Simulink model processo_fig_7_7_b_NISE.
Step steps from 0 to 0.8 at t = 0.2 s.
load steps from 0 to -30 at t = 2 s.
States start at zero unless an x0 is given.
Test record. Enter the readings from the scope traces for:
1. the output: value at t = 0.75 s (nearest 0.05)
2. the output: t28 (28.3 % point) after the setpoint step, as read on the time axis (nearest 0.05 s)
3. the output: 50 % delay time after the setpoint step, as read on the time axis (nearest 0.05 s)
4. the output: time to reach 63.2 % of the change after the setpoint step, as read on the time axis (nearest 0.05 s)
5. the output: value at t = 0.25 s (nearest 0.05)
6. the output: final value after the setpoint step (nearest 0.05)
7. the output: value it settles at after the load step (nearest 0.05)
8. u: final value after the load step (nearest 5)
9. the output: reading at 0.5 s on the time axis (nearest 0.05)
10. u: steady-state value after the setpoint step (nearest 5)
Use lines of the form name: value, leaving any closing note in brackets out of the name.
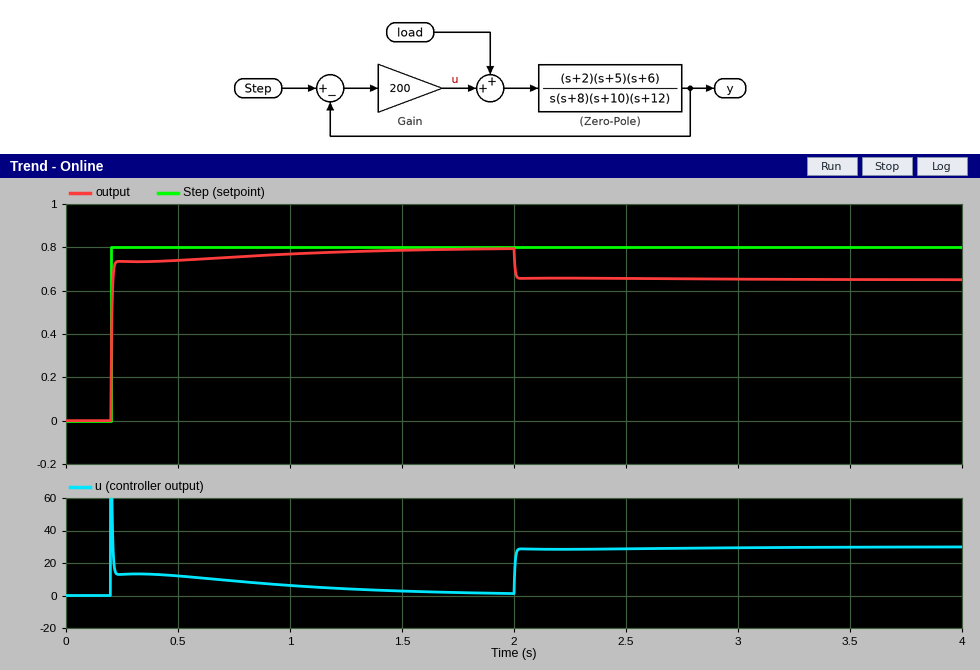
the output: value at t = 0.75 s: 0.75
the output: t28 (28.3 % point) after the setpoint step, as read on the time axis: 0.20 s
the output: 50 % delay time after the setpoint step, as read on the time axis: 0.20 s
the output: time to reach 63.2 % of the change after the setpoint step, as read on the time axis: 0.20 s
the output: value at t = 0.25 s: 0.75
the output: final value after the setpoint step: 0.80
the output: value it settles at after the load step: 0.65
u: final value after the load step: 30
the output: reading at 0.5 s on the time axis: 0.75
u: steady-state value after the setpoint step: 0
